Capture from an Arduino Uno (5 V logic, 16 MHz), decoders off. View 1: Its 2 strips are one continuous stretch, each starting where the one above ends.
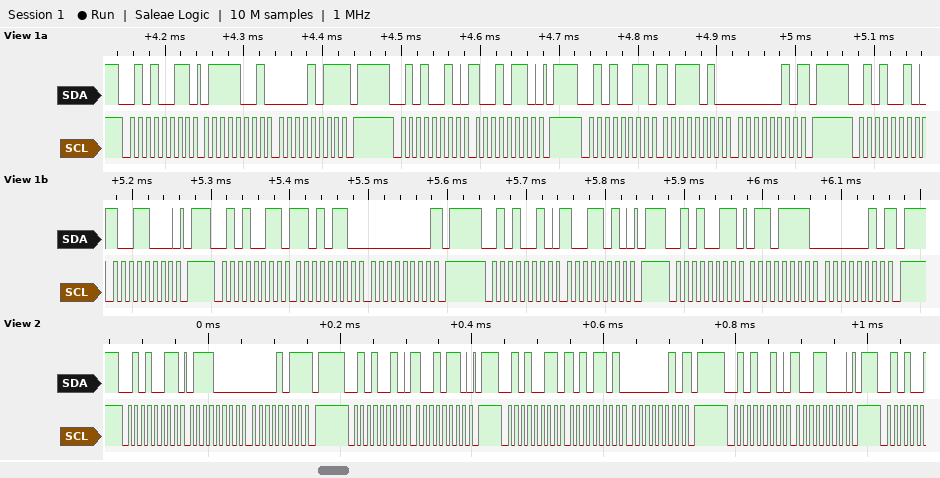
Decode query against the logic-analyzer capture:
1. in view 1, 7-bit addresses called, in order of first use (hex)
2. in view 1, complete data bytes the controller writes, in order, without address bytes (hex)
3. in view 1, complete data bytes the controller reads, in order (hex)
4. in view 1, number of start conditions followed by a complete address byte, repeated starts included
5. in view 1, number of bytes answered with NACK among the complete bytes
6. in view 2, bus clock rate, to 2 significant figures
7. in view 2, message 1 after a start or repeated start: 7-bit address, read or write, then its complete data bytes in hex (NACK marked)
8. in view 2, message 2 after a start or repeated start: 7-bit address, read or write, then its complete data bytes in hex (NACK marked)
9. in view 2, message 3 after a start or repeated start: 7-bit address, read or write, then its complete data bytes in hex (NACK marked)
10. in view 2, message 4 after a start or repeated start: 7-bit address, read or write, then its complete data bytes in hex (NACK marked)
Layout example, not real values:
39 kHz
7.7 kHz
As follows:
0x29
96 98 9A
79 0B BA 02 D6 00 6F 02
7
4
100 kHz
0x29 read: 70 0B NACK
0x29 write: 96
0x29 read: AD 02 NACK
0x29 write: 98
